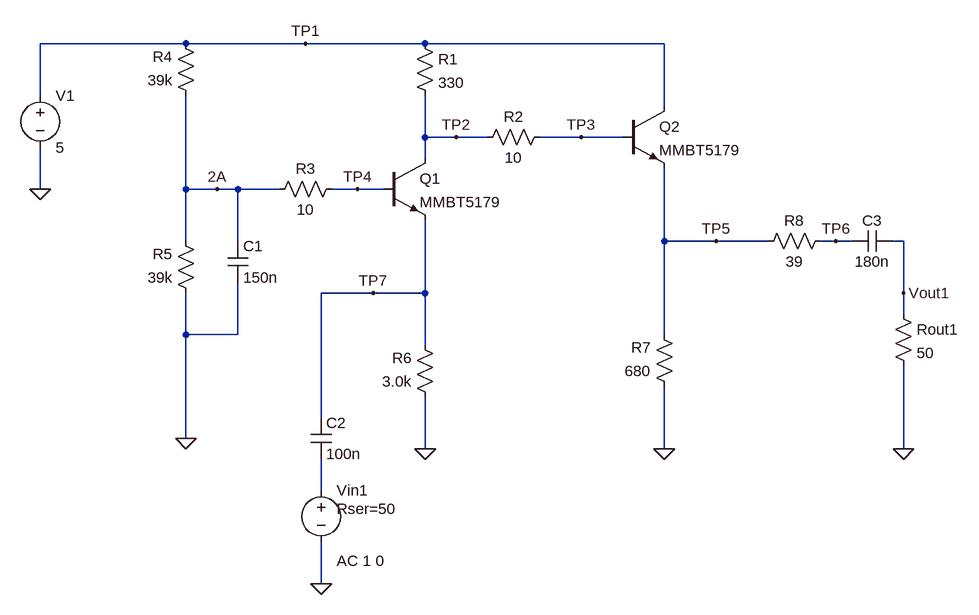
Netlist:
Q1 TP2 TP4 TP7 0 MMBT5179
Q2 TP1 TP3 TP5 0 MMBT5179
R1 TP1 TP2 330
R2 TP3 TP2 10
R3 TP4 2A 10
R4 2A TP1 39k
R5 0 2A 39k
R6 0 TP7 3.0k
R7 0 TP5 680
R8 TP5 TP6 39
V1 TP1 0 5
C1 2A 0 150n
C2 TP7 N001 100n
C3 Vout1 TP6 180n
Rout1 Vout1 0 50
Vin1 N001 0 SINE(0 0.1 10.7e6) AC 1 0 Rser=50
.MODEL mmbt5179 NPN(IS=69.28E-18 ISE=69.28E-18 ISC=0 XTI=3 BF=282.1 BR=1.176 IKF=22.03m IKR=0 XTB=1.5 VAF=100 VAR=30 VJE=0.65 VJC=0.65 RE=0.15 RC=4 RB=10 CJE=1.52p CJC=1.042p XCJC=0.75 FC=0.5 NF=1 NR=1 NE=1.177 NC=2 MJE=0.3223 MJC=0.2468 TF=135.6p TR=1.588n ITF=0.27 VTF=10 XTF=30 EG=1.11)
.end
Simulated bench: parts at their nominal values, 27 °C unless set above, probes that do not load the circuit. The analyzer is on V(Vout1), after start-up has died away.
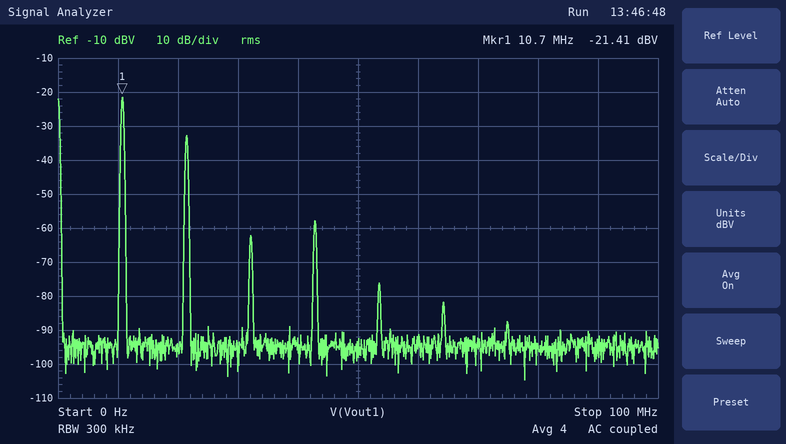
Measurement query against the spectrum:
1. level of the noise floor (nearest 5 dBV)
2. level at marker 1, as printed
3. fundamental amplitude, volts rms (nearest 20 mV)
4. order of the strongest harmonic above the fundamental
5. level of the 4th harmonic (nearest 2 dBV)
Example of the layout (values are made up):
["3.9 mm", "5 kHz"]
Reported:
["-95 dBV", "-21.41 dBV", "80 mV", "2", "-58 dBV"]
